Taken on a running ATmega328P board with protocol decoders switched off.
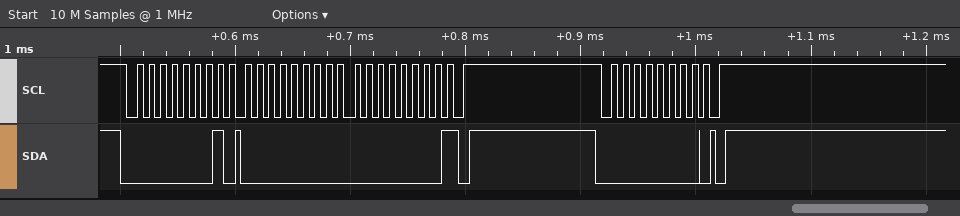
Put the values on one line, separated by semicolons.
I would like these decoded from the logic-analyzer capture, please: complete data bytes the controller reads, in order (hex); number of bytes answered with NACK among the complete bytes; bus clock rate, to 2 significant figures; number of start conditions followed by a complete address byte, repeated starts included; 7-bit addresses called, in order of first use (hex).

00 00; 1; 100 kHz; 2; 0x00
